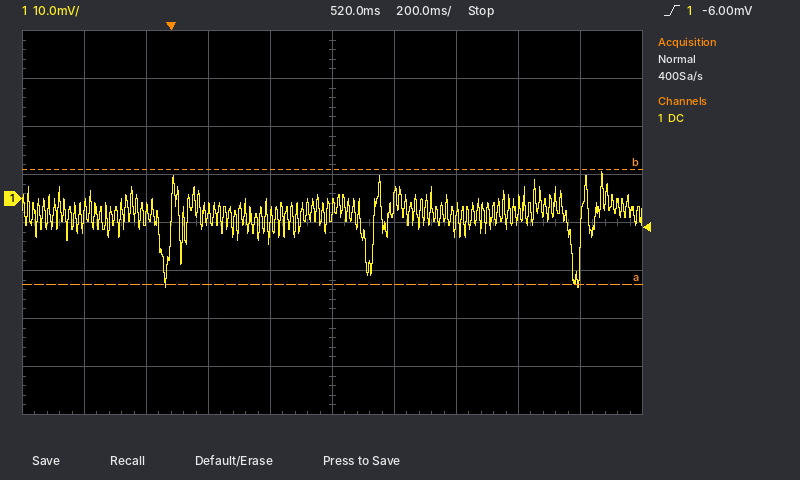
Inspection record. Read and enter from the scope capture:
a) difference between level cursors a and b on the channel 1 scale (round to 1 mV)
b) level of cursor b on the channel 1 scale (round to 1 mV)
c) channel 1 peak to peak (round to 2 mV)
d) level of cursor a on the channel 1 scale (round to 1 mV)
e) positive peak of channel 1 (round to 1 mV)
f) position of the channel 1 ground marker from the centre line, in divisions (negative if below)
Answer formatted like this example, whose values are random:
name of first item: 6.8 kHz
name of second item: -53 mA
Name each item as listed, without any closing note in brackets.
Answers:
difference between level cursors a and b on the channel 1 scale: 24 mV
level of cursor b on the channel 1 scale: 6 mV
channel 1 peak to peak: 24 mV
level of cursor a on the channel 1 scale: -18 mV
positive peak of channel 1: 6 mV
position of the channel 1 ground marker from the centre line, in divisions: +0.5 div
